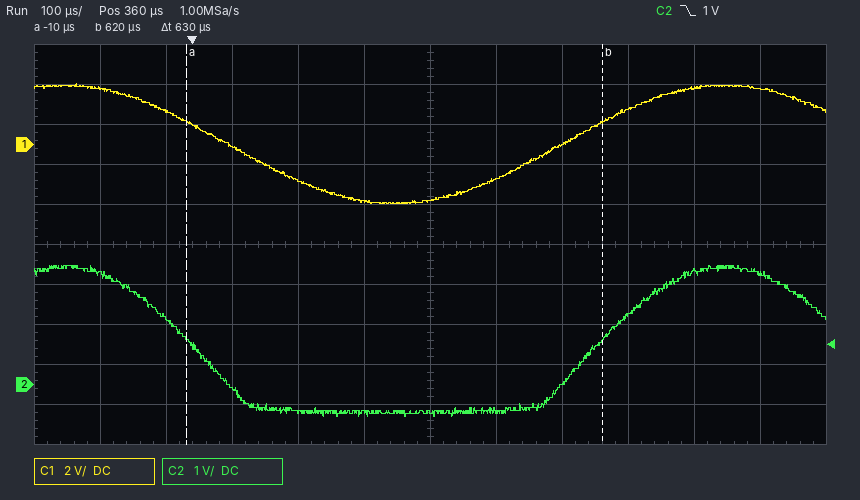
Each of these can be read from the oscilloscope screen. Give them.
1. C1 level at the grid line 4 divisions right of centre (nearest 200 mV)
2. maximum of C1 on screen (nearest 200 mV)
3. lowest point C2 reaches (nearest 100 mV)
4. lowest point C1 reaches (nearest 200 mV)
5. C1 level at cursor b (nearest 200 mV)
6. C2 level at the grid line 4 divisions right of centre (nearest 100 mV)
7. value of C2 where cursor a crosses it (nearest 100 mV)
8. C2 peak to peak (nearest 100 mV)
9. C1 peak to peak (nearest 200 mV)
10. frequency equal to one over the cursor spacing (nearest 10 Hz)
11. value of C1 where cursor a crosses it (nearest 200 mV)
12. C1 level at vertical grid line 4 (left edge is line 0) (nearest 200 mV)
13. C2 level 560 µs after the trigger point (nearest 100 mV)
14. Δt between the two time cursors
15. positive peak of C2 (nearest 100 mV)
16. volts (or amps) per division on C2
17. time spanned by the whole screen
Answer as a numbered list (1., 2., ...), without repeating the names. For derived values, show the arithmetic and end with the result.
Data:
1. 2.8 V
2. 3.0 V
3. -800 mV
4. -3.0 V
5. 1.2 V
6. 2.8 V
7. 1.1 V
8. 3.0 V − (-800 mV) = 3.8 V
9. 3.0 V − (-3.0 V) = 6.0 V
10. 1 / 630 µs ≈ 1.59 kHz
11. 1.2 V
12. -1.8 V
13. 0.0 V
14. 630 µs
15. 3.0 V
16. 1 V
17. 1.2 ms
